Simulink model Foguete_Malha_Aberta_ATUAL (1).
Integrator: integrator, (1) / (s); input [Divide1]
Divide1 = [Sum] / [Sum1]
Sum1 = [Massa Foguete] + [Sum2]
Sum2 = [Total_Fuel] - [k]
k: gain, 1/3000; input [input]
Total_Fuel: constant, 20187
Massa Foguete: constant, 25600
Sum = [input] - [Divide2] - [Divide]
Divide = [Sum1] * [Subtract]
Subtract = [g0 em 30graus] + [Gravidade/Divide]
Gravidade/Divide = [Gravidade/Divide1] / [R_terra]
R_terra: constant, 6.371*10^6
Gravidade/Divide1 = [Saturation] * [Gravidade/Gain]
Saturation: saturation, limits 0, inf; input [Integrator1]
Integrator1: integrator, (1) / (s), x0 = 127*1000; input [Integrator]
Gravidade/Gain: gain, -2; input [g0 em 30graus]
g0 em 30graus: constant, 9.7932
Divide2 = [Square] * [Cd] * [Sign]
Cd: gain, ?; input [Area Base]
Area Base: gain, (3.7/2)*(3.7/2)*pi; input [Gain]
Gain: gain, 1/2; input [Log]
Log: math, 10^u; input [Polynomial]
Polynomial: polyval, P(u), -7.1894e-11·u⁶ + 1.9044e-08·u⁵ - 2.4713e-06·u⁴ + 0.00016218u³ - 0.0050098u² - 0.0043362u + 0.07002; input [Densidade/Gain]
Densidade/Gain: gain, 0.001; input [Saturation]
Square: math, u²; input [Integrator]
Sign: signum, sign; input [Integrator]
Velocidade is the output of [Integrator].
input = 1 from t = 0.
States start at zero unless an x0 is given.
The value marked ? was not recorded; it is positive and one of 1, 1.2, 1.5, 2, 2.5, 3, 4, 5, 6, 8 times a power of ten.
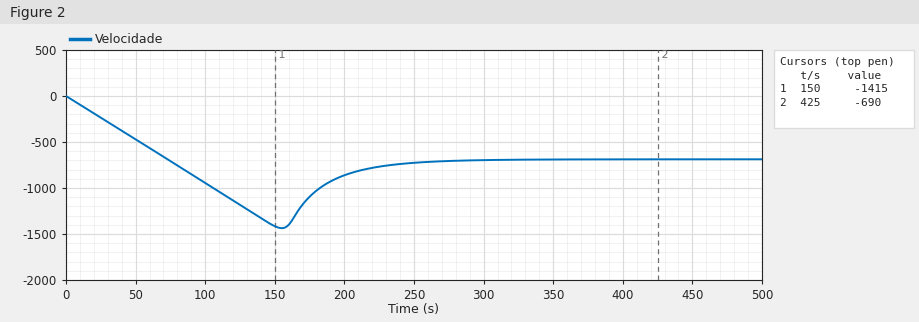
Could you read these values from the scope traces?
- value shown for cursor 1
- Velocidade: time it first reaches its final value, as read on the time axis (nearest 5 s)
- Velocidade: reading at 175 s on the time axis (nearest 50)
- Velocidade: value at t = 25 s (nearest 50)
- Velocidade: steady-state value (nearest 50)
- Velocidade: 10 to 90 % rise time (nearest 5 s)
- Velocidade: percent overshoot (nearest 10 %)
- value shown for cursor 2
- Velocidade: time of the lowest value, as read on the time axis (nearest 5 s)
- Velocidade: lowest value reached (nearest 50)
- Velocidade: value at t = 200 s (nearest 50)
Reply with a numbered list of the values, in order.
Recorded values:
1. -1415
2. 75 s
3. -1100
4. -250
5. -700
6. 60 s
7. 110 %
8. -690
9. 155 s
10. -1450
11. -850
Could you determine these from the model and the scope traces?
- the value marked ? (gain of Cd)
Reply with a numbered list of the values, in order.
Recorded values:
1. 0.15
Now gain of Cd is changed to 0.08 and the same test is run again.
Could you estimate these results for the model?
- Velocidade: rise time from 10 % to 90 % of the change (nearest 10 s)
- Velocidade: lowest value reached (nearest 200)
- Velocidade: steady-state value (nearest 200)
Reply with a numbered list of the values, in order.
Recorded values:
1. 80 s
2. -1400
3. -1000
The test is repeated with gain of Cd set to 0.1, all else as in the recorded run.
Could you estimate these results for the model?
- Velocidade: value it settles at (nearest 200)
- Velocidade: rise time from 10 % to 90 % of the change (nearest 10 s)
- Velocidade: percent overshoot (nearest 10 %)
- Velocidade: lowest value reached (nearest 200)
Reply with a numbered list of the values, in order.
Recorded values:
1. -800
2. 70 s
3. 70 %
4. -1400
